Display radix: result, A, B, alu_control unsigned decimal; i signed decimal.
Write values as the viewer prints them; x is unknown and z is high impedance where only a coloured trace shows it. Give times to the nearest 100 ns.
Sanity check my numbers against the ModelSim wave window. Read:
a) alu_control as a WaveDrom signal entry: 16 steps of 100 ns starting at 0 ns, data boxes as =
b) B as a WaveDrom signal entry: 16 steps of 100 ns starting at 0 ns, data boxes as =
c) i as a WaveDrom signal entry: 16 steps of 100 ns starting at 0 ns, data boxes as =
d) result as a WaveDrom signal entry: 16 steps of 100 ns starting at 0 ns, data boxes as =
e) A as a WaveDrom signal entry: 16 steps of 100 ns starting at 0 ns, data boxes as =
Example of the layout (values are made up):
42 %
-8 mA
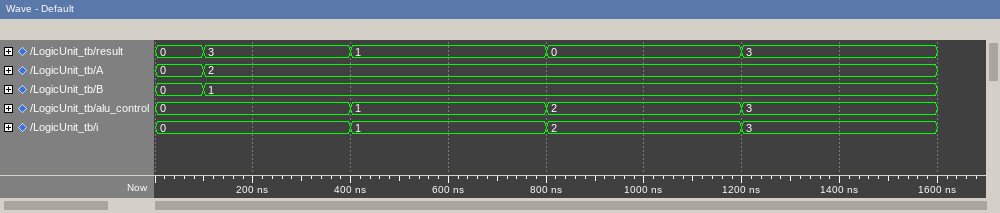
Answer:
{name: 'alu_control', wave: '=...=...=...=...', data: '0 1 2 3'}
{name: 'B', wave: '==..............', data: '0 1'}
{name: 'i', wave: '=...=...=...=...', data: '0 1 2 3'}
{name: 'result', wave: '==..=...=...=...', data: '0 3 1 0 3'}
{name: 'A', wave: '==..............', data: '0 2'}
